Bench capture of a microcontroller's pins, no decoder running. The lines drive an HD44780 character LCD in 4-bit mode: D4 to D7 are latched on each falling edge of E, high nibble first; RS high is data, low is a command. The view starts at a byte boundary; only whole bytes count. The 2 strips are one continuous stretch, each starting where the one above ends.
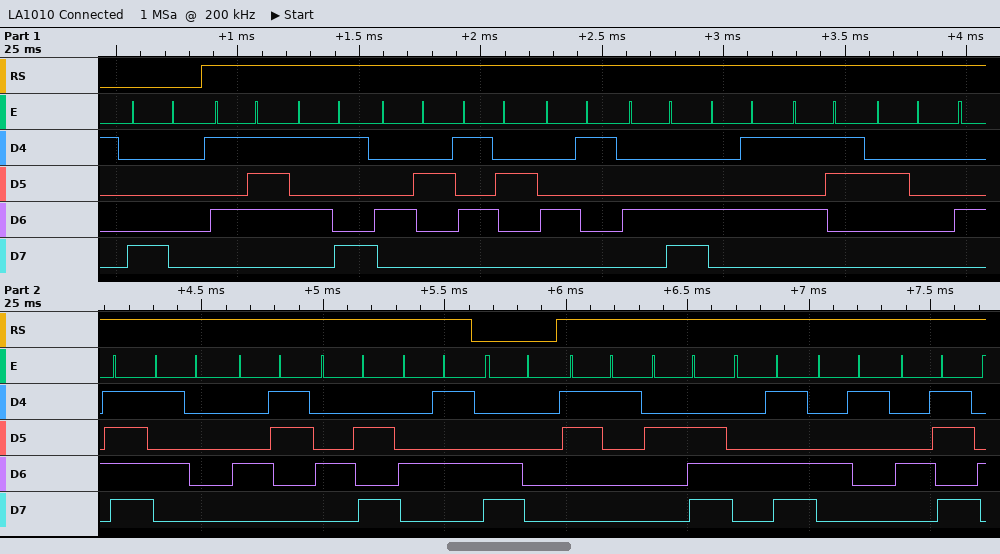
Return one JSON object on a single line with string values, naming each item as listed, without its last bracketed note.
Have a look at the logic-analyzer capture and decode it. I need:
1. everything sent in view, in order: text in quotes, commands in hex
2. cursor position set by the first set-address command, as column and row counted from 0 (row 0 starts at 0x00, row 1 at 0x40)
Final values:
{"everything sent in view, in order: text in quotes, commands in hex": "0x80 \"WYBRALES OPCJE\" 0xC0 \"1.MAK\"", "cursor position set by the first set-address command, as column and row counted from 0": "column 0, row 0"}
